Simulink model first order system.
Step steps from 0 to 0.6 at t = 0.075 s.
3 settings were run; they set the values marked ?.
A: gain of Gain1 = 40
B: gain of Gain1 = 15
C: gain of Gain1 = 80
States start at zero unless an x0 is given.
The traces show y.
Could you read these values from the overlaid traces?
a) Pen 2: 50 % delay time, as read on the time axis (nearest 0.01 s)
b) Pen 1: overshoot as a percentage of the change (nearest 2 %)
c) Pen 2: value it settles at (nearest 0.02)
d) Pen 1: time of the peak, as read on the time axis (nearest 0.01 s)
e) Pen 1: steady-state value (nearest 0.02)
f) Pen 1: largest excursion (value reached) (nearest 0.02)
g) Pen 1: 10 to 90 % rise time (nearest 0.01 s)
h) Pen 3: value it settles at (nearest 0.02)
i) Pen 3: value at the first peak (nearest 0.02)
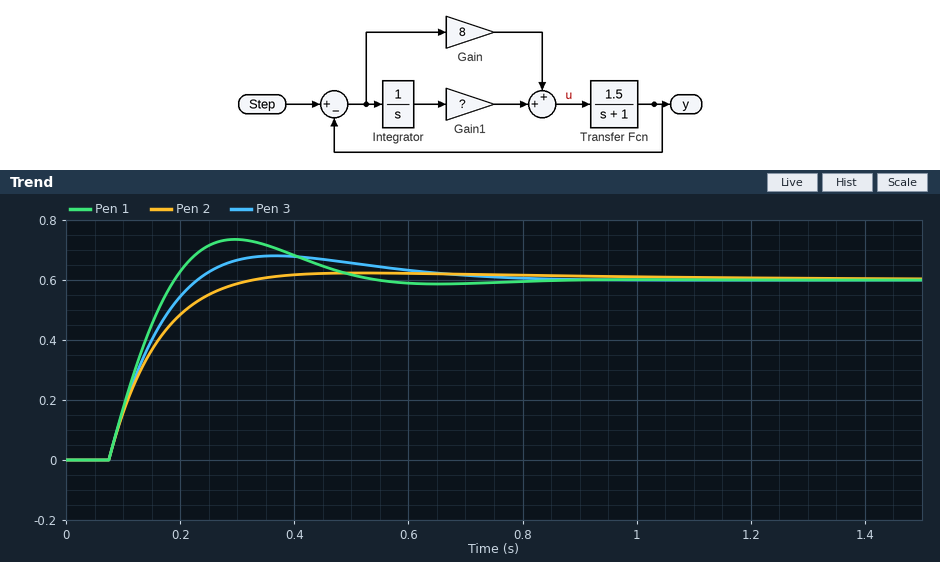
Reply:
0.13 s
22 %
0.60
0.30 s
0.60
0.74
0.09 s
0.60
0.68
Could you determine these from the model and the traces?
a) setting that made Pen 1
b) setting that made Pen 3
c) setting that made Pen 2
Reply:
C
A
B
